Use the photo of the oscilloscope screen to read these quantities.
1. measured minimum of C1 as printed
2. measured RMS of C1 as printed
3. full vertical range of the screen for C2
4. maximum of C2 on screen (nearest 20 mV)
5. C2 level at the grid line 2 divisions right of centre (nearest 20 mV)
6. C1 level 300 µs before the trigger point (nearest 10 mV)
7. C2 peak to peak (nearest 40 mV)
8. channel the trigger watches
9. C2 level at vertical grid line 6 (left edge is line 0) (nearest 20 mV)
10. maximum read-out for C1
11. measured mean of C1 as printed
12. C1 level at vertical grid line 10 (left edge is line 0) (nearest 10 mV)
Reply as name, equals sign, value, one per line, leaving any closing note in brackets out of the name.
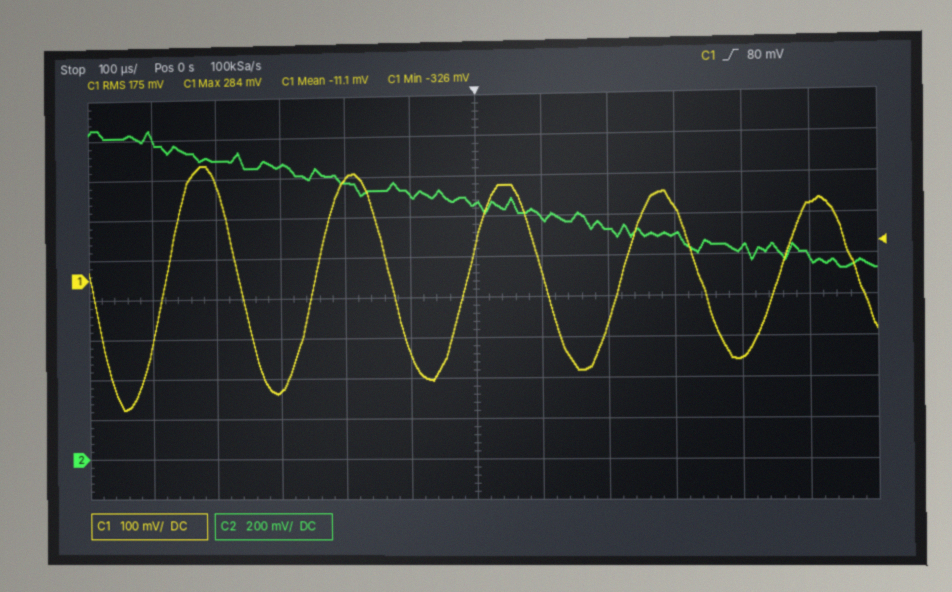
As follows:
measured minimum of C1 as printed = -326 mV
measured RMS of C1 as printed = 175 mV
full vertical range of the screen for C2 = 2 V
maximum of C2 on screen = 1.66 V
C2 level at the grid line 2 divisions right of centre = 1.14 V
C1 level 300 µs before the trigger point = -280 mV
C2 peak to peak = 720 mV
channel the trigger watches = C1
C2 level at vertical grid line 6 (left edge is line 0) = 1.26 V
maximum read-out for C1 = 284 mV
measured mean of C1 as printed = -11.1 mV
C1 level at vertical grid line 10 (left edge is line 0) = -200 mV
